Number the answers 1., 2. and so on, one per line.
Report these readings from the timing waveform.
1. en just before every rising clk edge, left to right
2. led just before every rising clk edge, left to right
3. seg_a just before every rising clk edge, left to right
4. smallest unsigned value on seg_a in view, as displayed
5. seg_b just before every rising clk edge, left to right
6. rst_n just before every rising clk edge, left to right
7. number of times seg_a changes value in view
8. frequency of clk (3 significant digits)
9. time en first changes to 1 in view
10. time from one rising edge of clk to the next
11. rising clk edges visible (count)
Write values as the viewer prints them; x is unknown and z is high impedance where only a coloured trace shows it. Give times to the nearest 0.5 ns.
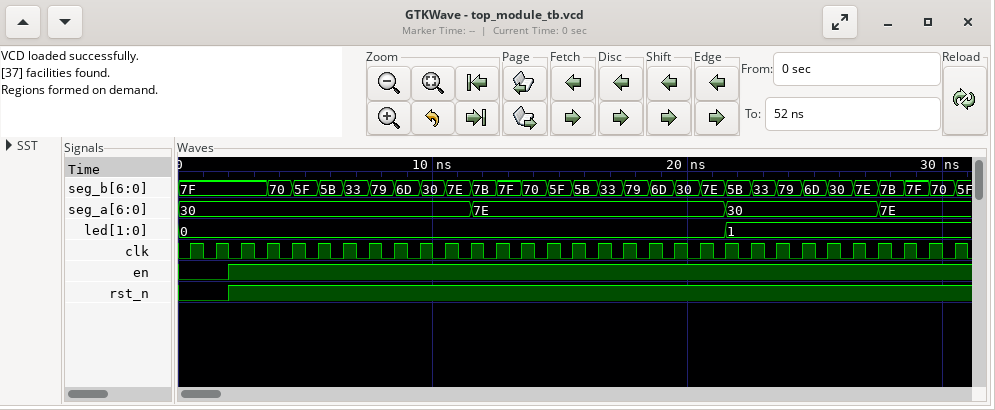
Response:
1. 0 0 1 1 1 1 1 1 1 1 1 1 1 1 1 1 1 1 1 1 1 1 1 1 1 1 1 1 1 1 1
2. 0, 0, 0, 0, 0, 0, 0, 0, 0, 0, 0, 0, 0, 0, 0, 0, 0, 0, 0, 0, 0, 0, 1, 1, 1, 1, 1, 1, 1, 1, 1
3. 30, 30, 30, 30, 30, 30, 30, 30, 30, 30, 30, 30, 7E, 7E, 7E, 7E, 7E, 7E, 7E, 7E, 7E, 7E, 30, 30, 30, 30, 30, 30, 7E, 7E, 7E
4. 30
5. 7F, 7F, 7F, 7F, 70, 5F, 5B, 33, 79, 6D, 30, 7E, 7B, 7F, 70, 5F, 5B, 33, 79, 6D, 30, 7E, 5B, 33, 79, 6D, 30, 7E, 7B, 7F, 70
6. 0 0 1 1 1 1 1 1 1 1 1 1 1 1 1 1 1 1 1 1 1 1 1 1 1 1 1 1 1 1 1
7. 3
8. 1.00 GHz
9. 2 ns
10. 1 ns
11. 31
